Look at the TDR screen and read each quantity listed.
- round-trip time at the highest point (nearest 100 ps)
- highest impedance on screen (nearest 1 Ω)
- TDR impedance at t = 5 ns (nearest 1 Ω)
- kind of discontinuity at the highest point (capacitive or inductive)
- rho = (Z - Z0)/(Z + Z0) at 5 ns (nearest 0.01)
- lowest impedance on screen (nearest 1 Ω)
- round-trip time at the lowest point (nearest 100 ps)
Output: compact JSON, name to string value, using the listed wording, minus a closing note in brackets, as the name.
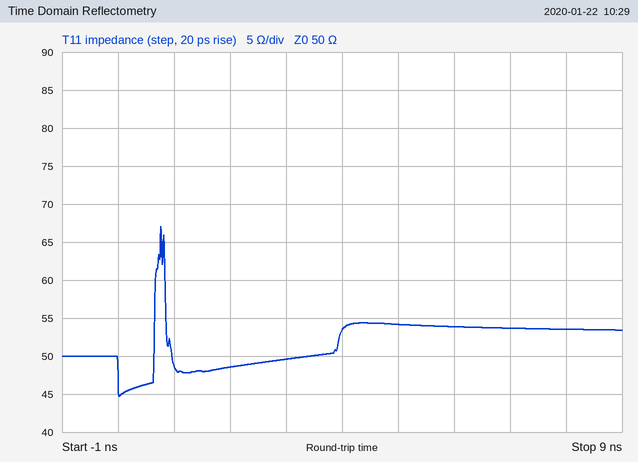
{"round-trip time at the highest point": "800 ps", "highest impedance on screen": "67 Ω", "TDR impedance at t = 5 ns": "54 Ω", "kind of discontinuity at the highest point": "inductive", "rho = (Z - Z0)/(Z + Z0) at 5 ns": "+0.04", "lowest impedance on screen": "45 Ω", "round-trip time at the lowest point": "0.0 ns"}
